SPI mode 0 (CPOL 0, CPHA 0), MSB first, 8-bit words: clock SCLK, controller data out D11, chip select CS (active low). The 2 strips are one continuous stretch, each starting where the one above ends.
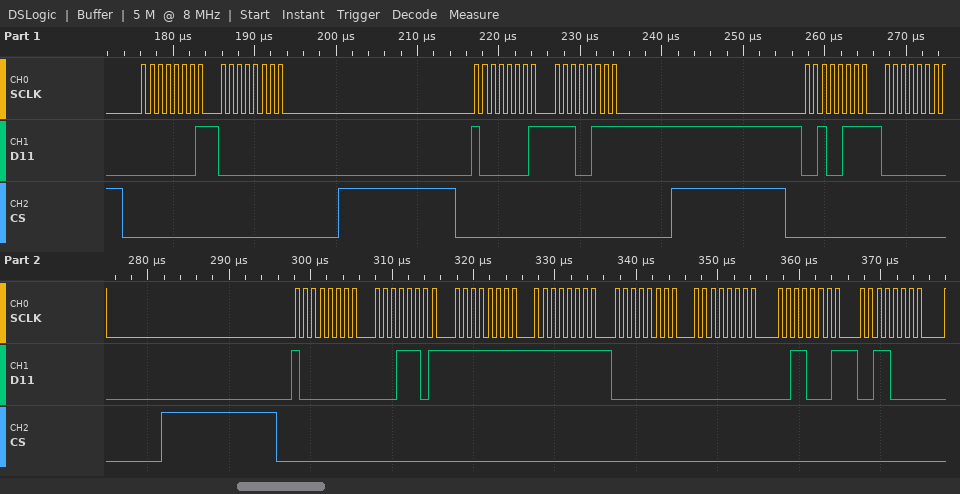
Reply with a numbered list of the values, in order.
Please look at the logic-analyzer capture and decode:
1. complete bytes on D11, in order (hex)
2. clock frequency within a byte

1. 01 00 81 E7 27 00 80 1D FF FF 00 00 31 30
2. 1 MHz
